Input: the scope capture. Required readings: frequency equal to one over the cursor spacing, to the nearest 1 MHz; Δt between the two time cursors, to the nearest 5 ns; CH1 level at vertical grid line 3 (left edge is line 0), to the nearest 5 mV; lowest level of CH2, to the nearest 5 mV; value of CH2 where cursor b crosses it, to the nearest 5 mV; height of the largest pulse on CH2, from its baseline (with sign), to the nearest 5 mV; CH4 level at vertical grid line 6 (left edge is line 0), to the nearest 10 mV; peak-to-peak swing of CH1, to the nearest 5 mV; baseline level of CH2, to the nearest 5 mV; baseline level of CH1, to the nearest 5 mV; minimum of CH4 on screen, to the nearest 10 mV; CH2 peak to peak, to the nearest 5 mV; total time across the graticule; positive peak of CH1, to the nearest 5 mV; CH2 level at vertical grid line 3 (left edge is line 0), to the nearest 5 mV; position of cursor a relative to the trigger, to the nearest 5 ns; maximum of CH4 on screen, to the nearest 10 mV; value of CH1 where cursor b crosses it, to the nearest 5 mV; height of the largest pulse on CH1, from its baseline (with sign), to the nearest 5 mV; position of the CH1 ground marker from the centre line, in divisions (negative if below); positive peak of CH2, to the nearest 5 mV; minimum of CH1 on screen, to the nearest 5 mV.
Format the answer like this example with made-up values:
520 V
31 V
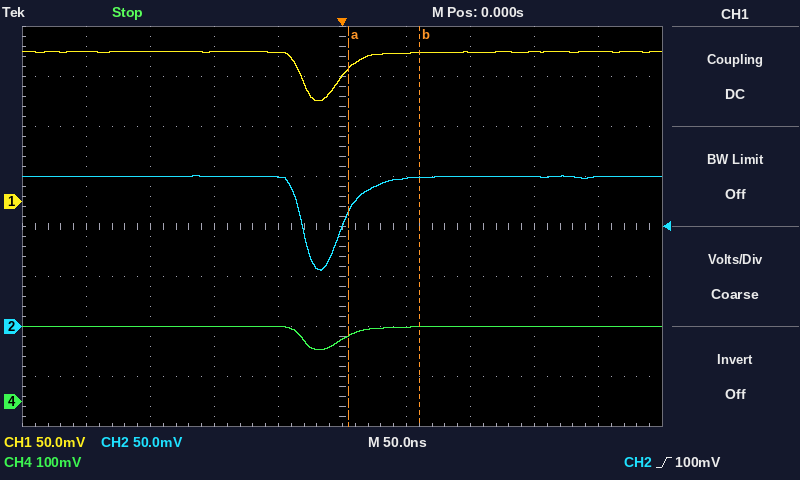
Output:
18 MHz
55 ns
150 mV
55 mV
150 mV
-95 mV
150 mV
50 mV
150 mV
150 mV
100 mV
95 mV
500 ns
150 mV
150 mV
+5 ns
150 mV
150 mV
-50 mV
+0.5 div
150 mV
100 mV
